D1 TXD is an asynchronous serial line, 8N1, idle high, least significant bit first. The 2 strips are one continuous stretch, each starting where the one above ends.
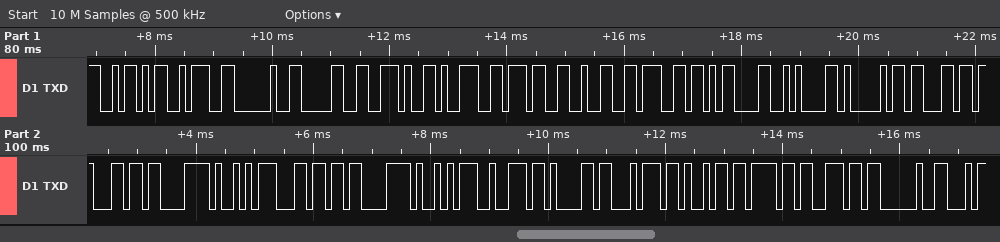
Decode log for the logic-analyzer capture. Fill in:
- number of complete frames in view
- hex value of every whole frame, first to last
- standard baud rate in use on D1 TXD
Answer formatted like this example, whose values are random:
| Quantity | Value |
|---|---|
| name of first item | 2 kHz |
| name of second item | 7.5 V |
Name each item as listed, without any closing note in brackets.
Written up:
| Quantity | Value |
|---|---|
| number of complete frames in view | 26 |
| hex value of every whole frame, first to last | 0x5A 0x3A 0x20 0x30 0x2E 0x39 0x37 0x32 0x67 0x0D 0x0A 0x41 0x63 0x63 0xC3 0xA9 0x6C 0xC3 0xA9 0x72 0x61 0x74 0x69 0x6F 0x6E 0x20 |
| standard baud rate in use on D1 TXD | 9600 baud |
